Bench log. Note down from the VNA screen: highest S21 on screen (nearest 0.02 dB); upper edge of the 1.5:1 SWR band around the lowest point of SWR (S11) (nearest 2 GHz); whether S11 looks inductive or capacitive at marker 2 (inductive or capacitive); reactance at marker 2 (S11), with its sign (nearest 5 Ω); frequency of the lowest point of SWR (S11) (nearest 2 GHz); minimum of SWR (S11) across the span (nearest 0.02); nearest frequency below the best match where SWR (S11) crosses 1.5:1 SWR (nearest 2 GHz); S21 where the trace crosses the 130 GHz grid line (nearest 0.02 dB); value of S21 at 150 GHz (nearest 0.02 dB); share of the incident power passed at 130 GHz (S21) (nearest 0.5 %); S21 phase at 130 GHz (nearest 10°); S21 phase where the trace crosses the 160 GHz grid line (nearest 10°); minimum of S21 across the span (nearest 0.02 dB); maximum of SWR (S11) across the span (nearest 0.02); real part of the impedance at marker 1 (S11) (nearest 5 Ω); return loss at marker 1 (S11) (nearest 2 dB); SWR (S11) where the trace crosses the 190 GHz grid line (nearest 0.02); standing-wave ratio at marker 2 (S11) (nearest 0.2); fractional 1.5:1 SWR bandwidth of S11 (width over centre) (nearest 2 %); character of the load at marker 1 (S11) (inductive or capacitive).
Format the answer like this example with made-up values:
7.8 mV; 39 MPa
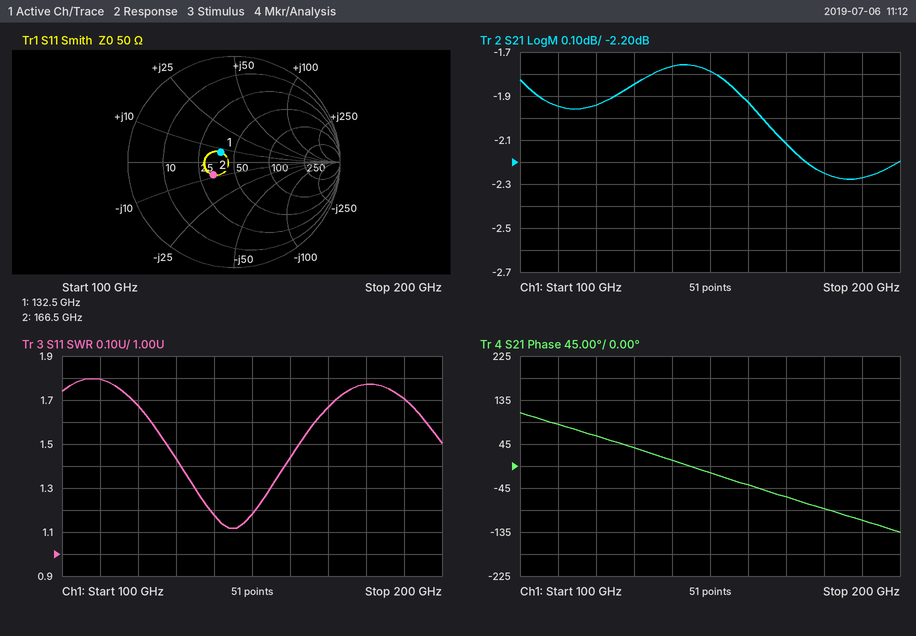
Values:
-1.76 dB; 162 GHz; capacitive; -10 Ω; 144 GHz; 1.12; 128 GHz; -1.84 dB; -1.78 dB; 65.5 %; 40°; -40°; -2.28 dB; 1.80; 40 Ω; 16 dB; 1.70; 1.6; 24 %; inductive
